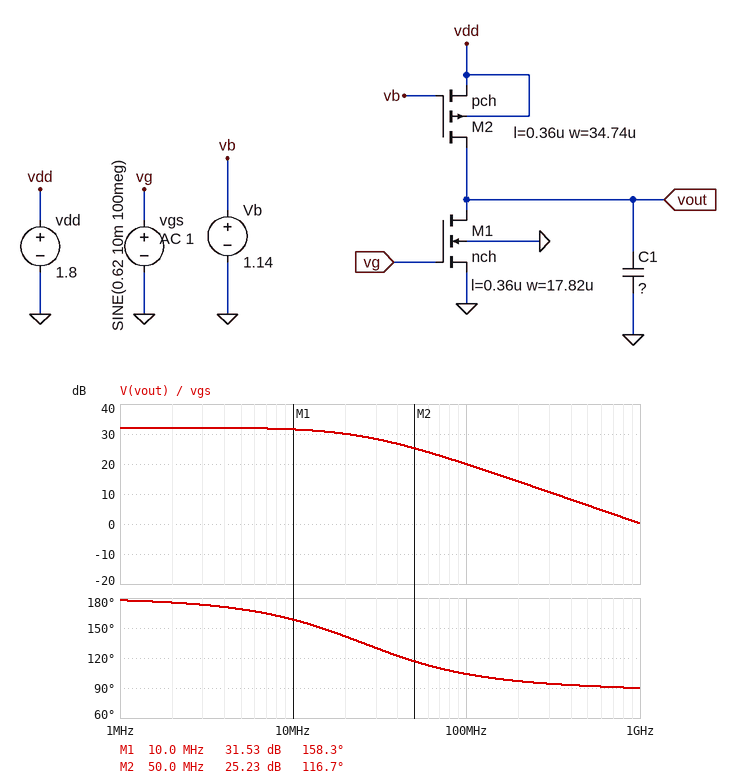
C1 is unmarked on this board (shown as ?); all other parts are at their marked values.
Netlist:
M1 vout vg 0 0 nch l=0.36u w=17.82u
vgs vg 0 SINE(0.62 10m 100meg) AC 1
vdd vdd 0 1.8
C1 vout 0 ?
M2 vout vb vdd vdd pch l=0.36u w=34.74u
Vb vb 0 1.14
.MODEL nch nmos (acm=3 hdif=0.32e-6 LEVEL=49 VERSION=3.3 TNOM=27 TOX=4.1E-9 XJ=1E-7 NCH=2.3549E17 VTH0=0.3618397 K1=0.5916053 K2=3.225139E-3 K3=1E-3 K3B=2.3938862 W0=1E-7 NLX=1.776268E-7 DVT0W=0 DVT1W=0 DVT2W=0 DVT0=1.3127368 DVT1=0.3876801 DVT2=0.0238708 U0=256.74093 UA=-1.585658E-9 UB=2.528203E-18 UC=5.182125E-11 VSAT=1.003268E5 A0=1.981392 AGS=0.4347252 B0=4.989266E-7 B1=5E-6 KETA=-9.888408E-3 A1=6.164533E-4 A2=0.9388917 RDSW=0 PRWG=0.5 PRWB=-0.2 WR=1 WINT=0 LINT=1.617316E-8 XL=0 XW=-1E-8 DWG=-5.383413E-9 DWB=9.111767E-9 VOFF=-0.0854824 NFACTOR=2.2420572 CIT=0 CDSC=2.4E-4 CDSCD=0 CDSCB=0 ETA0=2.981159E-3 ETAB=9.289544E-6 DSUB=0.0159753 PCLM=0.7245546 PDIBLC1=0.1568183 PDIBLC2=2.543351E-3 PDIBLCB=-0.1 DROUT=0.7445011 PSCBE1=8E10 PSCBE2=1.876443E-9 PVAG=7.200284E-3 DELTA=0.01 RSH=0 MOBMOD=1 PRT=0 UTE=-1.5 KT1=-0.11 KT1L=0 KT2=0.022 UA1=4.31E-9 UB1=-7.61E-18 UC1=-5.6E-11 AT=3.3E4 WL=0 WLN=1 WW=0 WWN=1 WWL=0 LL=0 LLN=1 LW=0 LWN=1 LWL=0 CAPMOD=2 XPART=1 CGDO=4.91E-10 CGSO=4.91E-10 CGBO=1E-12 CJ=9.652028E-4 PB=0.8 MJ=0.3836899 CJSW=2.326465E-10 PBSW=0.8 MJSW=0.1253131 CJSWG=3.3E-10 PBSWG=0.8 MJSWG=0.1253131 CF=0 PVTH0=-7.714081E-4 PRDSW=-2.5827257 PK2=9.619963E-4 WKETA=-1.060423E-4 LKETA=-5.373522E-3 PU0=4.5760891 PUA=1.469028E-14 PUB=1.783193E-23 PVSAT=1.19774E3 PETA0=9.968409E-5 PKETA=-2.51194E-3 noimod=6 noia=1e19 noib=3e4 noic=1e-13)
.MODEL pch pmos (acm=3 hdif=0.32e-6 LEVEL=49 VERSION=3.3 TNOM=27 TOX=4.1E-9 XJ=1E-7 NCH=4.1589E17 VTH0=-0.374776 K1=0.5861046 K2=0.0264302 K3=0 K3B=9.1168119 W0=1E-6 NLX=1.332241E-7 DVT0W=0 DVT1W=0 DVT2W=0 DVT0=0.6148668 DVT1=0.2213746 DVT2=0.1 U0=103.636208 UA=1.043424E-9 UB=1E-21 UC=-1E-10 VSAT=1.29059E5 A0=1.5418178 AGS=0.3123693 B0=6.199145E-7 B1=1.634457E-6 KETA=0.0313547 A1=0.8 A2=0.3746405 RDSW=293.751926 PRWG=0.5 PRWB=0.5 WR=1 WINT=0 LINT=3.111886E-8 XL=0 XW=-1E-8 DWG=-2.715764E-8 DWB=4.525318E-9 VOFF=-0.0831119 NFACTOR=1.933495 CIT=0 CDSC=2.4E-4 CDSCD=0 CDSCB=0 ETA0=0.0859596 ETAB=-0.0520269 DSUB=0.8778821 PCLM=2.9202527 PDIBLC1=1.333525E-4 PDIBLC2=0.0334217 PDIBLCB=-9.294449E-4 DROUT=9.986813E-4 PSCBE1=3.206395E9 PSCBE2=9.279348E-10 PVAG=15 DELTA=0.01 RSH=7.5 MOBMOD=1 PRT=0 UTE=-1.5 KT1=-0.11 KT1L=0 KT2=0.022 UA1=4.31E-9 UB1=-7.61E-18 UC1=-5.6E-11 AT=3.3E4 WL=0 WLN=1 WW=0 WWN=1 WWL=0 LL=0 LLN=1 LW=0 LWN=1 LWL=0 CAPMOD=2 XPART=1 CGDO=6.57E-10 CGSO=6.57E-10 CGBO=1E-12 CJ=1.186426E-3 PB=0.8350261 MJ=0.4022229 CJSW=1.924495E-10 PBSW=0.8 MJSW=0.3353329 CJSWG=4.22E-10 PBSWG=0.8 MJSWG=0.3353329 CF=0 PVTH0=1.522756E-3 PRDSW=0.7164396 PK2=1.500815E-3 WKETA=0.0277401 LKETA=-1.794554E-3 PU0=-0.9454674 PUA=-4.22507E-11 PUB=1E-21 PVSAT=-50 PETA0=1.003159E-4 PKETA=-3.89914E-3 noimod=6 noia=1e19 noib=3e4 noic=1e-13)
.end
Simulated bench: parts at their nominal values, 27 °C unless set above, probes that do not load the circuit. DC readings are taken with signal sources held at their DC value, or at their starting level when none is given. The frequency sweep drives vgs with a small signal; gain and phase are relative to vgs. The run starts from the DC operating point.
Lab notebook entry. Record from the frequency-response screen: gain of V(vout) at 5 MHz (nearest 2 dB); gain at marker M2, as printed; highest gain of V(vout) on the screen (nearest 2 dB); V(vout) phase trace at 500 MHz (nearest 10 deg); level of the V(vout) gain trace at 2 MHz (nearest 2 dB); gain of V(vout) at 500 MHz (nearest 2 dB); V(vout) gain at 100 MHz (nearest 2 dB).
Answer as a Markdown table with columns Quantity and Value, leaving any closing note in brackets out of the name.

| Quantity | Value |
|---|---|
| gain of V(vout) at 5 MHz | 32 dB |
| gain at marker M2, as printed | 25.23 dB |
| highest gain of V(vout) on the screen | 32 dB |
| V(vout) phase trace at 500 MHz | 90 deg |
| level of the V(vout) gain trace at 2 MHz | 32 dB |
| gain of V(vout) at 500 MHz | 6 dB |
| V(vout) gain at 100 MHz | 20 dB |
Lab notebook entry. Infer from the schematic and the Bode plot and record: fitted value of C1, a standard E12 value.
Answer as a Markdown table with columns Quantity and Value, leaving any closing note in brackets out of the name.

| Quantity | Value |
|---|---|
| fitted value of C1, a standard E12 value | 220 fF |
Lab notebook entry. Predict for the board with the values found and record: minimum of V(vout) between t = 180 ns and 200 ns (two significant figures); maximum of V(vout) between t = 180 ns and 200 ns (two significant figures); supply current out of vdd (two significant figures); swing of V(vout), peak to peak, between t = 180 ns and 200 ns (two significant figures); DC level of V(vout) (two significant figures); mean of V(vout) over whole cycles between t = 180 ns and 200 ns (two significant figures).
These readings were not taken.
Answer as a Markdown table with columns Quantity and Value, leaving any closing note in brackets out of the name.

| Quantity | Value |
|---|---|
| minimum of V(vout) between t = 180 ns and 200 ns | 960 mV |
| maximum of V(vout) between t = 180 ns and 200 ns | 1.2 V |
| supply current out of vdd | 160 µA |
| swing of V(vout), peak to peak, between t = 180 ns and 200 ns | 200 mV |
| DC level of V(vout) | 1.1 V |
| mean of V(vout) over whole cycles between t = 180 ns and 200 ns | 1.1 V |
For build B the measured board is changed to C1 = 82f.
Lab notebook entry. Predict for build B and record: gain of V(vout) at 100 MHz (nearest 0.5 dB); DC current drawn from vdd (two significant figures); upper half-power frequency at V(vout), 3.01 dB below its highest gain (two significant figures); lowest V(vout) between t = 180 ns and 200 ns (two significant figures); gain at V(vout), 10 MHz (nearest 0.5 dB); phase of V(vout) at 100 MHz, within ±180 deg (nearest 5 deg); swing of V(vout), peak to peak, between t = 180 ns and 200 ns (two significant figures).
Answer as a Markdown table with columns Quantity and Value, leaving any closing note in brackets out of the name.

| Quantity | Value |
|---|---|
| gain of V(vout) at 100 MHz | 24.5 dB |
| DC current drawn from vdd | 160 µA |
| upper half-power frequency at V(vout), 3.01 dB below its highest gain | 46 MHz |
| lowest V(vout) between t = 180 ns and 200 ns | 890 mV |
| gain at V(vout), 10 MHz | 32.0 dB |
| phase of V(vout) at 100 MHz, within ±180 deg | 115 deg |
| swing of V(vout), peak to peak, between t = 180 ns and 200 ns | 340 mV |
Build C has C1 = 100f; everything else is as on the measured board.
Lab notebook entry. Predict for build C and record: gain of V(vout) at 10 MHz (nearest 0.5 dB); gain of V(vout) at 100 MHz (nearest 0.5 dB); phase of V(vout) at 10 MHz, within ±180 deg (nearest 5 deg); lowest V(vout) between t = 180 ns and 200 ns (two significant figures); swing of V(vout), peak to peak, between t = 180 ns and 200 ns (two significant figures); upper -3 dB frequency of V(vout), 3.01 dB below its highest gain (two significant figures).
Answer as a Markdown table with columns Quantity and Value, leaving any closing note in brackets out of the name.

| Quantity | Value |
|---|---|
| gain of V(vout) at 10 MHz | 32.0 dB |
| gain of V(vout) at 100 MHz | 24.0 dB |
| phase of V(vout) at 10 MHz, within ±180 deg | 165 deg |
| lowest V(vout) between t = 180 ns and 200 ns | 910 mV |
| swing of V(vout), peak to peak, between t = 180 ns and 200 ns | 310 mV |
| upper -3 dB frequency of V(vout), 3.01 dB below its highest gain | 41 MHz |
